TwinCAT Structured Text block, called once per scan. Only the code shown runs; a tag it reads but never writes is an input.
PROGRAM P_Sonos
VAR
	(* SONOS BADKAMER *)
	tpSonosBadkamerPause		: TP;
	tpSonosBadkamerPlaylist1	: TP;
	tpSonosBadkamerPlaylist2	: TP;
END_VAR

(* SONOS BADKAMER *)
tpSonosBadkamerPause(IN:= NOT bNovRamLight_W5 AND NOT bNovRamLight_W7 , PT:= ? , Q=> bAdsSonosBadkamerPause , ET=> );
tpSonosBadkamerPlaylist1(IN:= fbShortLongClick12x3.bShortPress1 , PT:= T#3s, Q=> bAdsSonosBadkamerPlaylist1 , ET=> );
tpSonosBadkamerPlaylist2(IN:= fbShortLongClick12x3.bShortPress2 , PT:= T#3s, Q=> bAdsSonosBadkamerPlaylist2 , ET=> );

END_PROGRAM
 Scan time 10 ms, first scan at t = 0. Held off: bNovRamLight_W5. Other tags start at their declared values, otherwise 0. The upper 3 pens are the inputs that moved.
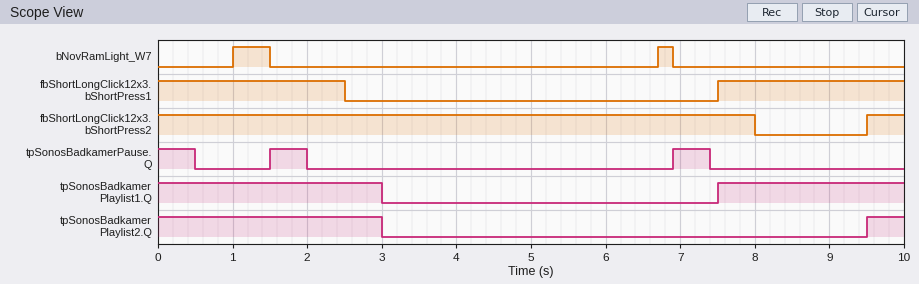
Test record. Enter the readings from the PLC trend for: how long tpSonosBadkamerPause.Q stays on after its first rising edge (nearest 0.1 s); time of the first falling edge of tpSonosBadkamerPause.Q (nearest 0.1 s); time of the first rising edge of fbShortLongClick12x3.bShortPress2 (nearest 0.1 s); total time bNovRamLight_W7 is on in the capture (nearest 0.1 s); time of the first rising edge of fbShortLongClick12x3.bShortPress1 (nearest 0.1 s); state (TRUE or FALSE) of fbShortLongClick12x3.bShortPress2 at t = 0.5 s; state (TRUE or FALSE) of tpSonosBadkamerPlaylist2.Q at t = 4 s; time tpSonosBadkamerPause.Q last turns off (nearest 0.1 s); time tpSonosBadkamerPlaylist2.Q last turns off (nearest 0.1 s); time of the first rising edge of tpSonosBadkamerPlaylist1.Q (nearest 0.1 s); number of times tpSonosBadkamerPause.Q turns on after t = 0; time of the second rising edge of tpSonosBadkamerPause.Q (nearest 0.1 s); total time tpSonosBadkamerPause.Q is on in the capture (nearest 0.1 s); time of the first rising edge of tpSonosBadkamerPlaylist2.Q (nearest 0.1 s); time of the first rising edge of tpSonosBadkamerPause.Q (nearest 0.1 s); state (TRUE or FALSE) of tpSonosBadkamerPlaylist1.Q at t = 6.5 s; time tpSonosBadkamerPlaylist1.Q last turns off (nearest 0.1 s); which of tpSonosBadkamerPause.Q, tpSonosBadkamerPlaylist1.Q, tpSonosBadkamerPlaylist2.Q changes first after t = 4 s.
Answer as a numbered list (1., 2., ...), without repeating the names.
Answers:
1. 0.5 s
2. 0.5 s
3. 9.5 s
4. 0.7 s
5. 7.5 s
6. TRUE
7. FALSE
8. 7.4 s
9. 3.0 s
10. 7.5 s
11. 2
12. 6.9 s
13. 1.5 s
14. 9.5 s
15. 1.5 s
16. FALSE
17. 3.0 s
18. tpSonosBadkamerPause.Q
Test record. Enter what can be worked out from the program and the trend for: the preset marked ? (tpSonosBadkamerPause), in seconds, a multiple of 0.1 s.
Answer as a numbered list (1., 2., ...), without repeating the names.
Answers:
1. 0.5 s
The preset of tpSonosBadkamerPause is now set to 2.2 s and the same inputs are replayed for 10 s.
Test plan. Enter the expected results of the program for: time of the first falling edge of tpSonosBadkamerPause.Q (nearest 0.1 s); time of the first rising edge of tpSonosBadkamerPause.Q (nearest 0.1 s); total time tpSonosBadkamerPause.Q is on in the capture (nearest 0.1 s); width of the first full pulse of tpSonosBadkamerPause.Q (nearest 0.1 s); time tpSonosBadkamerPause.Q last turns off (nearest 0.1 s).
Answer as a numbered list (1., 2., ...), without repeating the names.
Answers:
1. 2.2 s
2. 6.9 s
3. 4.4 s
4. 2.2 s
5. 9.1 s
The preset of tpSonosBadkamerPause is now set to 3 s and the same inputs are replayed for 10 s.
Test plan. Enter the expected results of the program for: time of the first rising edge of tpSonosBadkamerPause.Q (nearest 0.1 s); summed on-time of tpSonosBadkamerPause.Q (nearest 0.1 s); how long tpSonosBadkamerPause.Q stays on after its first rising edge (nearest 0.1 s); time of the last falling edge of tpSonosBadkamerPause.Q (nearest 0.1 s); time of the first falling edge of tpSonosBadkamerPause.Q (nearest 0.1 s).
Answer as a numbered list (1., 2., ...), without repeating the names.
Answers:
1. 6.9 s
2. 6.0 s
3. 3.0 s
4. 9.9 s
5. 3.0 s
